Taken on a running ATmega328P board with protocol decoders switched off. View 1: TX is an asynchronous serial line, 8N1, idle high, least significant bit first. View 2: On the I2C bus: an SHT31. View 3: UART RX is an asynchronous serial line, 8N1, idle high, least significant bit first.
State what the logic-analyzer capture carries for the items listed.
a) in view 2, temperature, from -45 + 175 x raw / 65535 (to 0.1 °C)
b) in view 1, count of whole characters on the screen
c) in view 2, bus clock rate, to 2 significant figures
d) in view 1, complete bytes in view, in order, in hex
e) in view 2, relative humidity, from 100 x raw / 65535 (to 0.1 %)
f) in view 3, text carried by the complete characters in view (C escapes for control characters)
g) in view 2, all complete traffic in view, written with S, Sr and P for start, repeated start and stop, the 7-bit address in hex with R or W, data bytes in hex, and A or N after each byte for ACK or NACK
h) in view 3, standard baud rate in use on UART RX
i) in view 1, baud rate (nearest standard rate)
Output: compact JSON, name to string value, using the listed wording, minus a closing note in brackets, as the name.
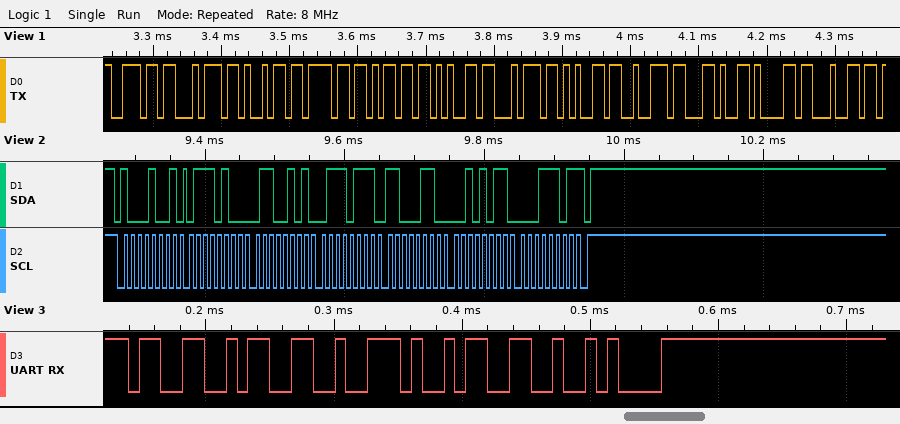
{"in view 2, temperature, from -45 + 175 x raw / 65535": "34.6 °C", "in view 1, count of whole characters on the screen": "12", "in view 2, bus clock rate, to 2 significant figures": "100 kHz", "in view 1, complete bytes in view, in order, in hex": "6E 74 69 6F 6D 65 74 65 72 2C 61 64", "in view 2, relative humidity, from 100 x raw / 65535": "77.4 %", "in view 3, text carried by the complete characters in view": "\"33.3\\n\"", "in view 2, all complete traffic in view, written with S, Sr and P for start, repeated start and stop, the 7-bit address in hex with R or W, data bytes in hex, and A or N after each byte for ACK or NACK": "S 44R A 74 A 65 A 77 A C6 A 2B A 1D N P", "in view 3, standard baud rate in use on UART RX": "115200 baud", "in view 1, baud rate": "115200 baud"}
